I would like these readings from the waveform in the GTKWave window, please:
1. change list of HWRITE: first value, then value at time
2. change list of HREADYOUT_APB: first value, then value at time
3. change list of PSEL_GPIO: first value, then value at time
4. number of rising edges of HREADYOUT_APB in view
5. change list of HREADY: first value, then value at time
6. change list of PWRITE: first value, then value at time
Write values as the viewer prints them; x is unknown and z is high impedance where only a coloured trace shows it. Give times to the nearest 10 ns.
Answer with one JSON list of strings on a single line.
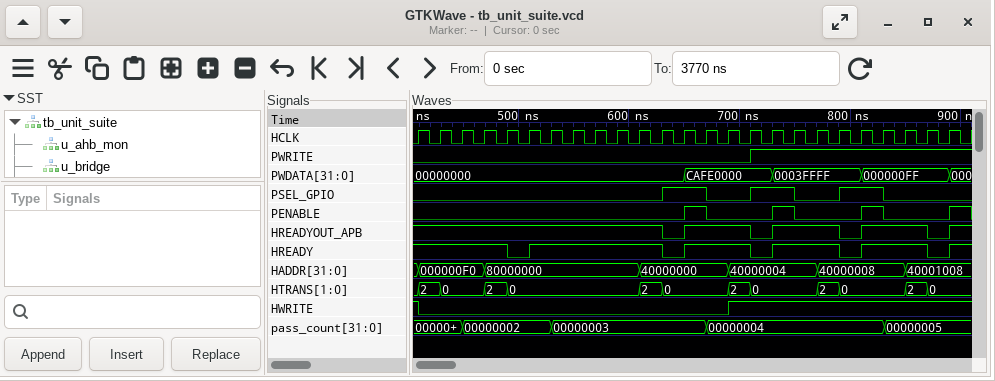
["1, 0 at 410 ns, 1 at 690 ns", "1, 0 at 630 ns, 1 at 650 ns, 0 at 710 ns, 1 at 730 ns, 0 at 790 ns, 1 at 810 ns, 0 at 870 ns, 1 at 890 ns", "0, 1 at 630 ns, 0 at 670 ns, 1 at 710 ns, 0 at 750 ns, 1 at 790 ns, 0 at 830 ns", "4", "1, 0 at 490 ns, 1 at 510 ns, 0 at 630 ns, 1 at 650 ns, 0 at 710 ns, 1 at 730 ns, 0 at 790 ns, 1 at 810 ns, 0 at 870 ns, 1 at 890 ns", "0, 1 at 710 ns"]
